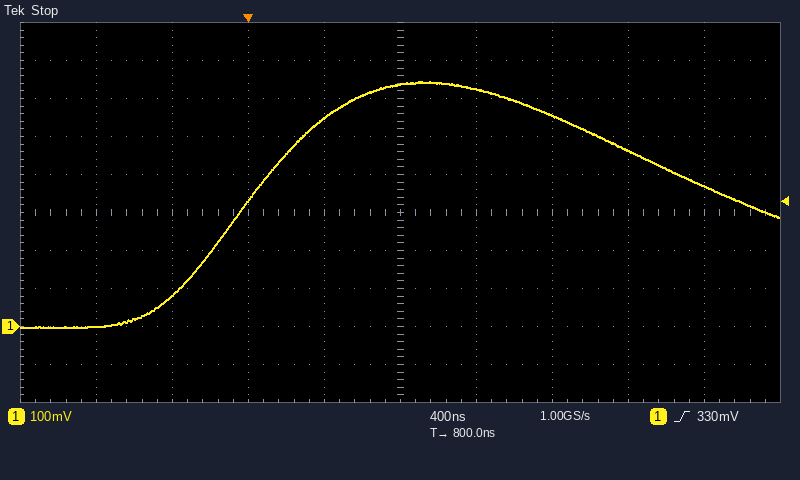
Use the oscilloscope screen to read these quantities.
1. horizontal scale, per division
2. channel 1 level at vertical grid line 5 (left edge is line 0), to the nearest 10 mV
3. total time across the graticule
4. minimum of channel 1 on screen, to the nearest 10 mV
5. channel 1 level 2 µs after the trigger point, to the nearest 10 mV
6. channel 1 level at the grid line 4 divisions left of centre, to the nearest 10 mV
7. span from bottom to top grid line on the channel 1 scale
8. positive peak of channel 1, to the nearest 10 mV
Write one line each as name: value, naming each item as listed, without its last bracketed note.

horizontal scale, per division: 400 ns
channel 1 level at vertical grid line 5 (left edge is line 0), to the nearest 10 mV: 640 mV
total time across the graticule: 4 µs
minimum of channel 1 on screen, to the nearest 10 mV: 0 mV
channel 1 level 2 µs after the trigger point, to the nearest 10 mV: 460 mV
channel 1 level at the grid line 4 divisions left of centre, to the nearest 10 mV: 0 mV
span from bottom to top grid line on the channel 1 scale: 1 V
positive peak of channel 1, to the nearest 10 mV: 640 mV
